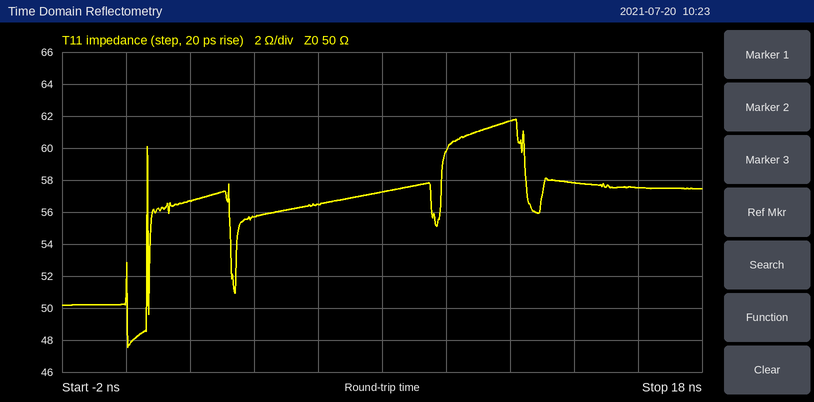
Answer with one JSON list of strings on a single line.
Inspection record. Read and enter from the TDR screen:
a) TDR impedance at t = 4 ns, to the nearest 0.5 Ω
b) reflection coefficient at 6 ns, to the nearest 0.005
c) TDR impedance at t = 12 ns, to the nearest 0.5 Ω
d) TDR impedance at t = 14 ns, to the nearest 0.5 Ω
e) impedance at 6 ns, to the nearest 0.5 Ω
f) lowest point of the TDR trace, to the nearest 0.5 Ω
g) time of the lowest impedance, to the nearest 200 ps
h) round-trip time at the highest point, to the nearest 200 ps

["55.5 Ω", "+0.060", "61.5 Ω", "58.0 Ω", "56.5 Ω", "47.5 Ω", "0.0 ns", "12.2 ns"]
